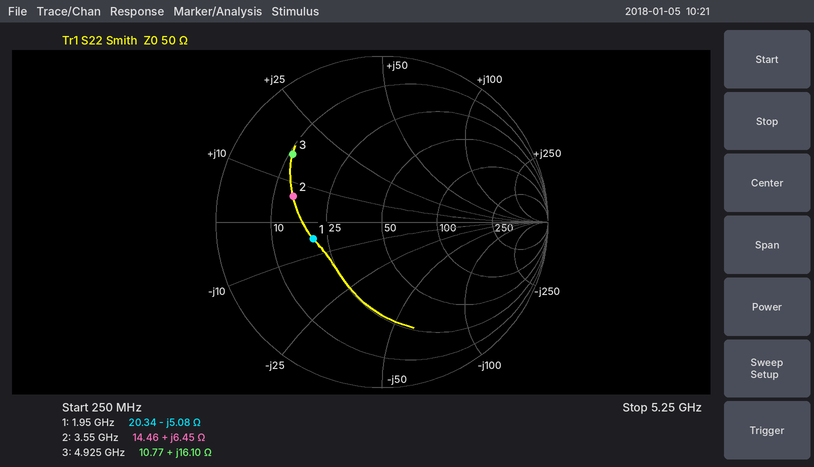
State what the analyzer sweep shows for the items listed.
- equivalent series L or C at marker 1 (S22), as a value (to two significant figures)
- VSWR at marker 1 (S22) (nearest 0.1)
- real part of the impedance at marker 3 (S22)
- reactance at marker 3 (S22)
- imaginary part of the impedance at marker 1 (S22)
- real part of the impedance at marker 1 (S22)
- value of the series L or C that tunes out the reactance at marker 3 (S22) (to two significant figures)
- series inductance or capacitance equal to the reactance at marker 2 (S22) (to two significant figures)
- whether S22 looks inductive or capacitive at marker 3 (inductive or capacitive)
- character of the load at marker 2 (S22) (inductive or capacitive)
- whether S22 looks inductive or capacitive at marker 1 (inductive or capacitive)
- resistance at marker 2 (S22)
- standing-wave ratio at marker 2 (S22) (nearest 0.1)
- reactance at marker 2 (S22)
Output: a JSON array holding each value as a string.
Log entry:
["16 pF", "2.5", "10.77 Ω", "+16.10 Ω", "-5.08 Ω", "20.34 Ω", "2.0 pF", "290 pH", "inductive", "inductive", "capacitive", "14.46 Ω", "3.5", "+6.45 Ω"]
